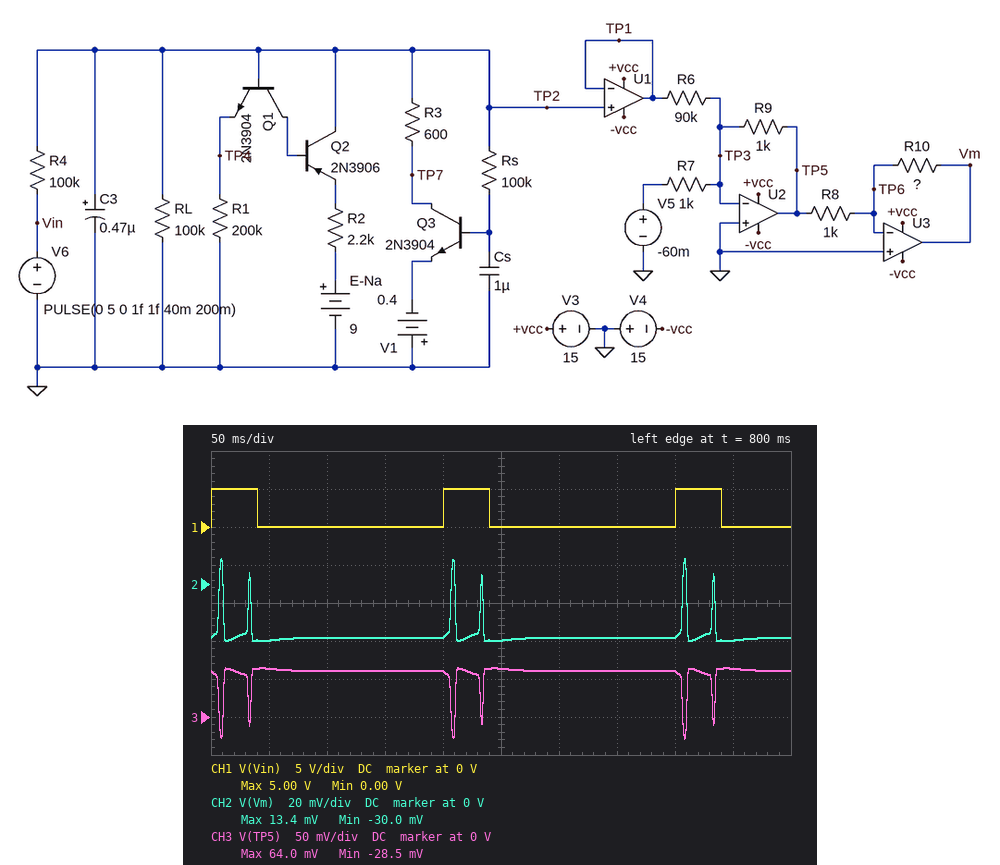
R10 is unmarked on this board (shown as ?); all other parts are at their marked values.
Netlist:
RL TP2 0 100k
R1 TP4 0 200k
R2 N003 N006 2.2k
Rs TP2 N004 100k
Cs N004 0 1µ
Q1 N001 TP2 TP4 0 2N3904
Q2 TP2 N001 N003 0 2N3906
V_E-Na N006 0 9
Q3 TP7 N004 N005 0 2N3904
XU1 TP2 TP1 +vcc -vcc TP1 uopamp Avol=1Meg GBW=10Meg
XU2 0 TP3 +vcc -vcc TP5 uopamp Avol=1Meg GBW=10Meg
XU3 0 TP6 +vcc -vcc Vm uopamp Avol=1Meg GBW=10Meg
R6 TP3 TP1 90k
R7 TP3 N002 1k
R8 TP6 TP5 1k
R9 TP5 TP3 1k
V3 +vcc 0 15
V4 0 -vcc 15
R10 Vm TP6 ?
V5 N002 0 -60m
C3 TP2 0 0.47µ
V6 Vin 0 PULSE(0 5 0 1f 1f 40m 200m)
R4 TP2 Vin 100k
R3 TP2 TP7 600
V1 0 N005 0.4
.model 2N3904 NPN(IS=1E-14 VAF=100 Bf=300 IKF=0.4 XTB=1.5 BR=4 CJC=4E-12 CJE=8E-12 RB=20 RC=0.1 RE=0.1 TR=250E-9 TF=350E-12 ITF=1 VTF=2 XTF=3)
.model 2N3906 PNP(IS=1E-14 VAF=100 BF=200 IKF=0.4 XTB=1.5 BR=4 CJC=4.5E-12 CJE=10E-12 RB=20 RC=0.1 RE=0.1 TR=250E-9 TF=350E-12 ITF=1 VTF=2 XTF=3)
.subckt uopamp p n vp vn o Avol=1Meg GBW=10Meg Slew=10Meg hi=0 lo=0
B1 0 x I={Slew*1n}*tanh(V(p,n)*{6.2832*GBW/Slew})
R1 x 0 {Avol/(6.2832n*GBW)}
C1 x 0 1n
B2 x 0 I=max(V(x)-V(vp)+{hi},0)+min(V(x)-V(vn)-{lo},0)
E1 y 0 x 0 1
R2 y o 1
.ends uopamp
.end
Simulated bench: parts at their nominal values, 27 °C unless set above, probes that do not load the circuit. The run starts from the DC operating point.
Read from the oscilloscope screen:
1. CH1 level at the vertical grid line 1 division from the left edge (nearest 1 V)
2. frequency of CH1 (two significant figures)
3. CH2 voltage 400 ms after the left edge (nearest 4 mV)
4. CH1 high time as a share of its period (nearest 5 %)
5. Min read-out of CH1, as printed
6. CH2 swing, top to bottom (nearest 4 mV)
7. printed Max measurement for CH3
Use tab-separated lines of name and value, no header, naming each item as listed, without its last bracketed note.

CH1 level at the vertical grid line 1 division from the left edge	0 V
frequency of CH1	5.0 Hz
CH2 voltage 400 ms after the left edge	-28 mV
CH1 high time as a share of its period	20 %
Min read-out of CH1, as printed	0.00 V
CH2 swing, top to bottom	44 mV
printed Max measurement for CH3	64.0 mV
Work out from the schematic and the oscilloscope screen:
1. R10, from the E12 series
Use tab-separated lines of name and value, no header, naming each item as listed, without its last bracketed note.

R10, from the E12 series	470 Ω
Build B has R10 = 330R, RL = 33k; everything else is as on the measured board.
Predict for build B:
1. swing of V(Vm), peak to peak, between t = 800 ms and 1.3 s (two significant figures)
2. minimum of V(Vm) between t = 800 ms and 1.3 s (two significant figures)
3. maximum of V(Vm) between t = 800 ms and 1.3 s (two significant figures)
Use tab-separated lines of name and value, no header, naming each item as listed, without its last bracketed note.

swing of V(Vm), peak to peak, between t = 800 ms and 1.3 s	29 mV
minimum of V(Vm) between t = 800 ms and 1.3 s	-21 mV
maximum of V(Vm) between t = 800 ms and 1.3 s	8.2 mV
